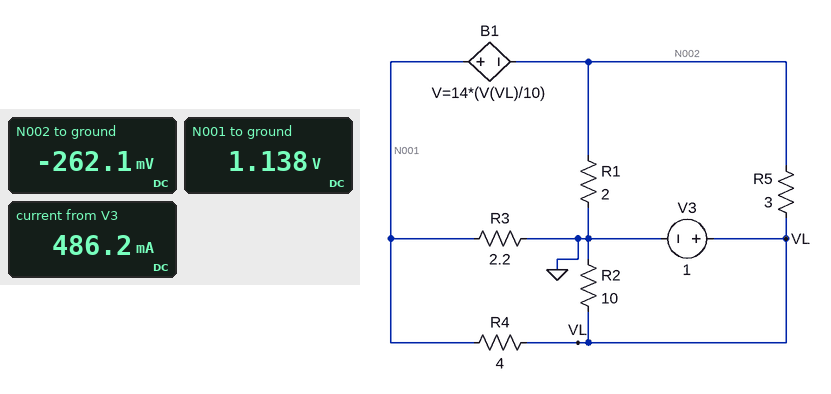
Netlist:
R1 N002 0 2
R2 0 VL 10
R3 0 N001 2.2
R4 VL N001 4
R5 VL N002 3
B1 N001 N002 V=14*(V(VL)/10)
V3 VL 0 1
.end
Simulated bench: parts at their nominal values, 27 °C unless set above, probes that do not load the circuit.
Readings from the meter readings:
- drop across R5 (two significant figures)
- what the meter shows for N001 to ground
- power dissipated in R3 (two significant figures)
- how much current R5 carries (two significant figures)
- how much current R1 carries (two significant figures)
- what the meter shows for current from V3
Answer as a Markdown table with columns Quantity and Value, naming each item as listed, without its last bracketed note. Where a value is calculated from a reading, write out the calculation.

| Quantity | Value |
|---|---|
| drop across R5 | 1 V - (-262.1 mV) = 1.3 V |
| what the meter shows for N001 to ground | 1.138 V |
| power dissipated in R3 | (1.138 V)^2 / 2.2 Ω = 590 mW |
| how much current R5 carries | (1 V - (-262.1 mV)) / 3 Ω = 420 mA |
| how much current R1 carries | (0 V - (-262.1 mV)) / 2 Ω = 130 mA |
| what the meter shows for current from V3 | 486.2 mA |
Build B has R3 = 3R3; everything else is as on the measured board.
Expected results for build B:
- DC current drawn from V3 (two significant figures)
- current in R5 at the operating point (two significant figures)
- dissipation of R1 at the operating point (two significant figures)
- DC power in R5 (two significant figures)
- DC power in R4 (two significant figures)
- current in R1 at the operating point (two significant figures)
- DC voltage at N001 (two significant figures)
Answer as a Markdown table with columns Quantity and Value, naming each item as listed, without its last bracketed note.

| Quantity | Value |
|---|---|
| DC current drawn from V3 | 410 mA |
| current in R5 at the operating point | 380 mA |
| dissipation of R1 at the operating point | 9.5 mW |
| DC power in R5 | 430 mW |
| DC power in R4 | 17 mW |
| current in R1 at the operating point | 69 mA |
| DC voltage at N001 | 1.3 V |
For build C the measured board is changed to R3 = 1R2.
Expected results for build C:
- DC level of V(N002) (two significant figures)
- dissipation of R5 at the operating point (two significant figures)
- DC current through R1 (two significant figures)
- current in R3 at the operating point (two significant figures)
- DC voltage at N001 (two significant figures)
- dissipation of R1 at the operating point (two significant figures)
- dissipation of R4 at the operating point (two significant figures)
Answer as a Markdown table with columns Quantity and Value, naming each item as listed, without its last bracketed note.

| Quantity | Value |
|---|---|
| DC level of V(N002) | -490 mV |
| dissipation of R5 at the operating point | 740 mW |
| DC current through R1 | 240 mA |
| current in R3 at the operating point | 760 mA |
| DC voltage at N001 | 910 mV |
| dissipation of R1 at the operating point | 120 mW |
| dissipation of R4 at the operating point | 1.9 mW |
